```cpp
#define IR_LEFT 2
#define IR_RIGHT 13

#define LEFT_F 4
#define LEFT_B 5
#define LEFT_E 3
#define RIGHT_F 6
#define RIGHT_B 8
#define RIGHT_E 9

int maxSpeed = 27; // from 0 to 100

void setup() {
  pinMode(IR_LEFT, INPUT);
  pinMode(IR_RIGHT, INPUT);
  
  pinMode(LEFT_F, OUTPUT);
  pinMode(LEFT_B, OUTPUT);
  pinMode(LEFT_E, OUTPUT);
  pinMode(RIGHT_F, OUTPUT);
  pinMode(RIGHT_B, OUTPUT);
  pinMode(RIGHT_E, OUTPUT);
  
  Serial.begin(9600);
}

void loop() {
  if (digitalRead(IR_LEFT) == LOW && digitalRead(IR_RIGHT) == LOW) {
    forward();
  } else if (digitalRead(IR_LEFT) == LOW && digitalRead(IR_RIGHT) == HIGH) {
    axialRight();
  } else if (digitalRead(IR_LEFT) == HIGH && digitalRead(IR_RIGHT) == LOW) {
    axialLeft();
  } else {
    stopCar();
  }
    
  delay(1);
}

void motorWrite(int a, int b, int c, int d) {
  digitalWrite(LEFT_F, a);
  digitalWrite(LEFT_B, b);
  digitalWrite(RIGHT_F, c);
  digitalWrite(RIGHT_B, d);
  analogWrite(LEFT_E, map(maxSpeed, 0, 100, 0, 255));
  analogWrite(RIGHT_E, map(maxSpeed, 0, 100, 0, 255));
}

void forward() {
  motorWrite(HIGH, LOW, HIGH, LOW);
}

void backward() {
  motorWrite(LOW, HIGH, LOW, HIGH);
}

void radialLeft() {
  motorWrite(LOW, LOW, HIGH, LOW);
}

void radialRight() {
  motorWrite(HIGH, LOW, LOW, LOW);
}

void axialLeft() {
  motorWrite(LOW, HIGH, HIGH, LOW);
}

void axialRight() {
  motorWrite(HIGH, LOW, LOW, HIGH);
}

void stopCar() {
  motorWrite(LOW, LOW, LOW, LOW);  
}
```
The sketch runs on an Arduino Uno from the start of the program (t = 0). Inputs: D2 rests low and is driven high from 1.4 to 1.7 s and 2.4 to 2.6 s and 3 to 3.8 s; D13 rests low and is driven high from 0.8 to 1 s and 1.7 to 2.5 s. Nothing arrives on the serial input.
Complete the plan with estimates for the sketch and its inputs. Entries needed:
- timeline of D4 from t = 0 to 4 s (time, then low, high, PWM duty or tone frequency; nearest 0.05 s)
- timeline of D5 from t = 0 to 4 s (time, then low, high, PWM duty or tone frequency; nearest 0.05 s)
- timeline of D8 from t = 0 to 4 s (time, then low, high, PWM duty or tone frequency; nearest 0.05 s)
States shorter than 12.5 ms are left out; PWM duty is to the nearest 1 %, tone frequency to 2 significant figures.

0 s high; 1.4 s low; 1.7 s high; 2.4 s low; 2.6 s high; 3 s low; 3.8 s high
0 s low; 1.4 s high; 1.7 s low; 2.5 s high; 2.6 s low; 3 s high; 3.8 s low
0 s low; 0.8 s high; 1 s low; 1.7 s high; 2.4 s low
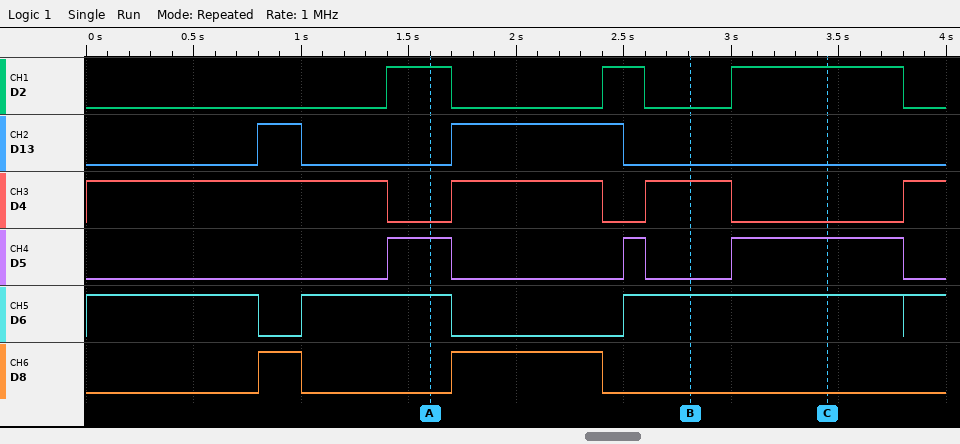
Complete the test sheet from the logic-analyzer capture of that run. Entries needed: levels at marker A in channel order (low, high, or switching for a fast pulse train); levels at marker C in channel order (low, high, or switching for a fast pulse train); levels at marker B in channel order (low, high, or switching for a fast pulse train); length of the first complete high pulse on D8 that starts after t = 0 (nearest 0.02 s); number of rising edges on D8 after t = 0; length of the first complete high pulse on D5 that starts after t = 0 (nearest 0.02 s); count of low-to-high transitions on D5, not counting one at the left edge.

D2 high, D13 low, D4 low, D5 high, D6 high, D8 low
D2 high, D13 low, D4 low, D5 high, D6 high, D8 low
D2 low, D13 low, D4 high, D5 low, D6 high, D8 low
0.20 s
2
0.30 s
3
